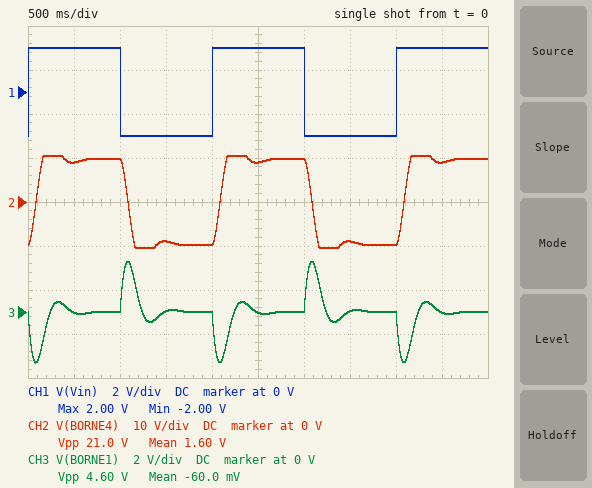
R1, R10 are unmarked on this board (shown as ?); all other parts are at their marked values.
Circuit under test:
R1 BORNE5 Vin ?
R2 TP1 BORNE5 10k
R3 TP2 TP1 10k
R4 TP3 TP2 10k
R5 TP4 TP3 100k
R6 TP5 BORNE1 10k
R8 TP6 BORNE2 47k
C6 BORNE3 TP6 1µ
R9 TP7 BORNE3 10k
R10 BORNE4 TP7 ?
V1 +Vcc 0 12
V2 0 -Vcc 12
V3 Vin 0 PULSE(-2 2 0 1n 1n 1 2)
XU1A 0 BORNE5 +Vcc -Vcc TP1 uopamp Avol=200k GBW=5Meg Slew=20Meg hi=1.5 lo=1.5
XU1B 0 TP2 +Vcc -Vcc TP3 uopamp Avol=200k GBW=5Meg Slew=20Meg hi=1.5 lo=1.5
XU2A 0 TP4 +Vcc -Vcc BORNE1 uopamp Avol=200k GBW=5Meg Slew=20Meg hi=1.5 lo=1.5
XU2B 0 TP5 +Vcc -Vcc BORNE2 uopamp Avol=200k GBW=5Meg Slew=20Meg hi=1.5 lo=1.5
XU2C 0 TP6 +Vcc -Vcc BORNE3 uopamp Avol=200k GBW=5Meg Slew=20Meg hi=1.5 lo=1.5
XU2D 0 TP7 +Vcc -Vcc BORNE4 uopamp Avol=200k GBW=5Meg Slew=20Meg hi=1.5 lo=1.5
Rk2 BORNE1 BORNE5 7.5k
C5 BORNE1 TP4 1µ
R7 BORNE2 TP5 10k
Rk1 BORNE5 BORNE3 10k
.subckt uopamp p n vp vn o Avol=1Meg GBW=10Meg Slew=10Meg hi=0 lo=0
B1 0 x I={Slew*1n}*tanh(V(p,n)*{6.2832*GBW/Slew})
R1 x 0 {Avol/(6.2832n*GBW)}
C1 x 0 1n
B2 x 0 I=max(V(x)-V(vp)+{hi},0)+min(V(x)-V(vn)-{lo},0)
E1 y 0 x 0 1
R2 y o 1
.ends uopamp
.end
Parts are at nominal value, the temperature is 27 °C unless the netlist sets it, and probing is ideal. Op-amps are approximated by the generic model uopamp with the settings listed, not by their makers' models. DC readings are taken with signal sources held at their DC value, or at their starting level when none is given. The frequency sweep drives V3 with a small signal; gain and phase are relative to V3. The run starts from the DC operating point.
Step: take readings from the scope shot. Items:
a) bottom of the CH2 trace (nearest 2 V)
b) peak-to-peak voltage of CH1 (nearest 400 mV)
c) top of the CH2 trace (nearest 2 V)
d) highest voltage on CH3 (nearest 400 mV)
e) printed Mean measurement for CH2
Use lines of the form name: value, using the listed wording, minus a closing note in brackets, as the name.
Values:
bottom of the CH2 trace: -10 V
peak-to-peak voltage of CH1: 4.0 V
top of the CH2 trace: 10 V
highest voltage on CH3: 2.4 V
printed Mean measurement for CH2: 1.60 V
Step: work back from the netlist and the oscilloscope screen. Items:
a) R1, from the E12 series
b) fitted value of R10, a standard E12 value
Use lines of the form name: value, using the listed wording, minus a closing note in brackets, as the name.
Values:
R1, from the E12 series: 6.8 kΩ
fitted value of R10, a standard E12 value: 33 kΩ
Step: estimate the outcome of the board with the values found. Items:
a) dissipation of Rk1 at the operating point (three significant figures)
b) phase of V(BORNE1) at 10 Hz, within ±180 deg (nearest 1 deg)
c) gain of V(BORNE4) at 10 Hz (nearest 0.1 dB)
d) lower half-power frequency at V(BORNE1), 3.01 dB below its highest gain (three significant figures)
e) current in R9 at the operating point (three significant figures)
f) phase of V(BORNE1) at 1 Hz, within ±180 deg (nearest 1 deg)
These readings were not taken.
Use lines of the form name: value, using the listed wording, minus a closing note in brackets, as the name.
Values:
dissipation of Rk1 at the operating point: 865 µW
phase of V(BORNE1) at 10 Hz, within ±180 deg: 103 deg
gain of V(BORNE4) at 10 Hz: -11.4 dB
lower half-power frequency at V(BORNE1), 3.01 dB below its highest gain: 1.49 Hz
current in R9 at the operating point: 294 µA
phase of V(BORNE1) at 1 Hz, within ±180 deg: -116 deg
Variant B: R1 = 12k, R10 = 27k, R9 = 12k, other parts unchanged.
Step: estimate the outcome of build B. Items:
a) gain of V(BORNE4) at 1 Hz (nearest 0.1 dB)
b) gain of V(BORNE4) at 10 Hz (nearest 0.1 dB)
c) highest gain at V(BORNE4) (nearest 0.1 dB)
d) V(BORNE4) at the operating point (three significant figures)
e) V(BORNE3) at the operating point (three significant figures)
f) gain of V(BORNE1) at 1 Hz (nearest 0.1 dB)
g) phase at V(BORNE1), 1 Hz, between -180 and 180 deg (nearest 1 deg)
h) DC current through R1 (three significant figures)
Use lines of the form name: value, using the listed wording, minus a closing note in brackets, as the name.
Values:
gain of V(BORNE4) at 1 Hz: 6.3 dB
gain of V(BORNE4) at 10 Hz: -19.6 dB
highest gain at V(BORNE4): 7.3 dB
V(BORNE4) at the operating point: -3.75 V
V(BORNE3) at the operating point: 1.67 V
gain of V(BORNE1) at 1 Hz: -11.3 dB
phase at V(BORNE1), 1 Hz, between -180 and 180 deg: -116 deg
DC current through R1: 167 µA
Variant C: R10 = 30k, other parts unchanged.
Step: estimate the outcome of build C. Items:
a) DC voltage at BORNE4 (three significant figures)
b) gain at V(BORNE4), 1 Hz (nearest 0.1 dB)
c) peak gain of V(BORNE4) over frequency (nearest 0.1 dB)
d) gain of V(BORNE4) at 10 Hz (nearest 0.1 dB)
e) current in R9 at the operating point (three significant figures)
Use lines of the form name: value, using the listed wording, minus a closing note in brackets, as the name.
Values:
DC voltage at BORNE4: -8.82 V
gain at V(BORNE4), 1 Hz: 13.8 dB
peak gain of V(BORNE4) over frequency: 14.7 dB
gain of V(BORNE4) at 10 Hz: -12.2 dB
current in R9 at the operating point: 294 µA
